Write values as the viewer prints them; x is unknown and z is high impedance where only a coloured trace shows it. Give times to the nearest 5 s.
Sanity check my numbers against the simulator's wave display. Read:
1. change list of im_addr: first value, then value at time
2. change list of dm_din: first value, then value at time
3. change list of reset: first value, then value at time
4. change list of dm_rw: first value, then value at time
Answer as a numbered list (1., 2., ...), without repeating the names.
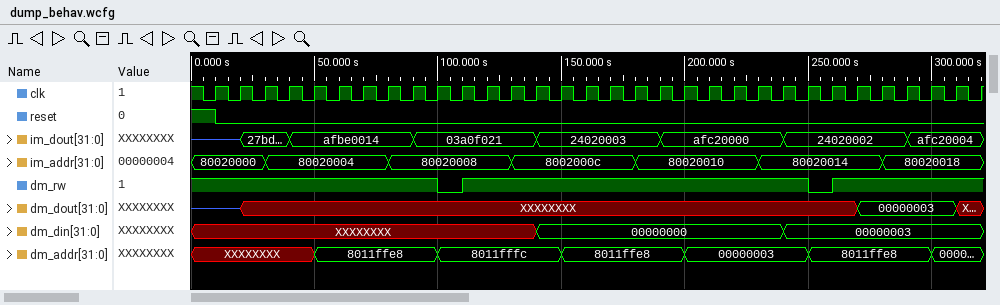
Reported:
1. 80020000, 80020004 at 30 s, 80020008 at 80 s, 8002000c at 130 s, 80020010 at 180 s, 80020014 at 230 s, 80020018 at 280 s
2. XXXXXXXX, 00000000 at 140 s, 00000003 at 240 s
3. 1, 0 at 10 s
4. 1, 0 at 100 s, 1 at 110 s, 0 at 250 s, 1 at 260 s
